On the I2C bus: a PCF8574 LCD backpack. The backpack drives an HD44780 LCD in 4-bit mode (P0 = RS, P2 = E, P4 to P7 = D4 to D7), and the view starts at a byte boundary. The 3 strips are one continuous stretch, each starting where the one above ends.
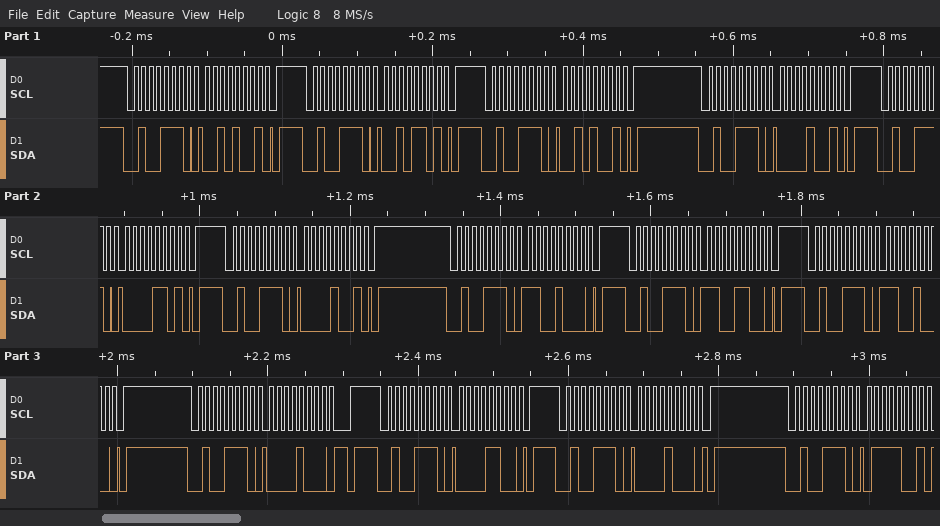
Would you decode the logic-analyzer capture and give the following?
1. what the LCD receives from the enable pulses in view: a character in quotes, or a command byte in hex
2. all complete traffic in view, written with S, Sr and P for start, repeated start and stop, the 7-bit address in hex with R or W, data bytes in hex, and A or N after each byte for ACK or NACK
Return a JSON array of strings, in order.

["' ' 0xC0", "S 27W A 29 A P S 27W A 2D A P S 27W A 29 A P S 27W A 09 A P S 27W A 0D A P S 27W A 09 A P S 27W A C8 A P S 27W A CC A P S 27W A C8 A P S 27W A 08 A P S 27W A 0C A P S 27W A 08 A P S 27W A 79 A"]
